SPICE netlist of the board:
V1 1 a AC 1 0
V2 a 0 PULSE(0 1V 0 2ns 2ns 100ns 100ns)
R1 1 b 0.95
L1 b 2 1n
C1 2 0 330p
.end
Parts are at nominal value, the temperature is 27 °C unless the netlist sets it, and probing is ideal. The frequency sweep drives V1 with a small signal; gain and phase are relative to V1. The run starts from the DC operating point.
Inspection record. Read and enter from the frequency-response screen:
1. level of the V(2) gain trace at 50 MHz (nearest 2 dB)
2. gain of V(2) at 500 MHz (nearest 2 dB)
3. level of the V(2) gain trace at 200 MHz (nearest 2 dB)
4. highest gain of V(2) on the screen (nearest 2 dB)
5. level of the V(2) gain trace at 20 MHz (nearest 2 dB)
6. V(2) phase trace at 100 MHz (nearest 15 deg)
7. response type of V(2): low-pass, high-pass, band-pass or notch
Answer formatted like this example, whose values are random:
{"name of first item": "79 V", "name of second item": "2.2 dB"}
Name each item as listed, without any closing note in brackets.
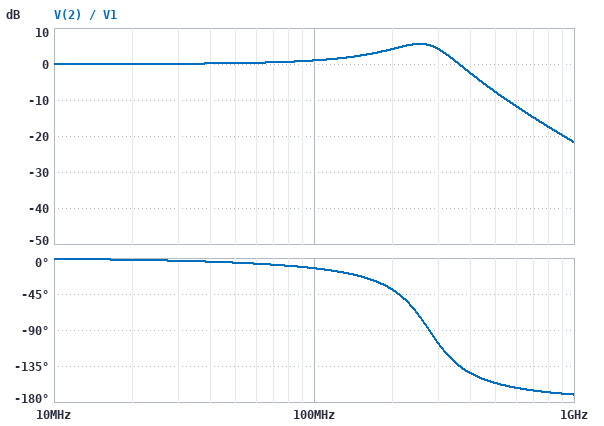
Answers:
{"level of the V(2) gain trace at 50 MHz": "0 dB", "gain of V(2) at 500 MHz": "-8 dB", "level of the V(2) gain trace at 200 MHz": "4 dB", "highest gain of V(2) on the screen": "6 dB", "level of the V(2) gain trace at 20 MHz": "0 dB", "V(2) phase trace at 100 MHz": "-15 deg", "response type of V(2): low-pass, high-pass, band-pass or notch": "low-pass"}
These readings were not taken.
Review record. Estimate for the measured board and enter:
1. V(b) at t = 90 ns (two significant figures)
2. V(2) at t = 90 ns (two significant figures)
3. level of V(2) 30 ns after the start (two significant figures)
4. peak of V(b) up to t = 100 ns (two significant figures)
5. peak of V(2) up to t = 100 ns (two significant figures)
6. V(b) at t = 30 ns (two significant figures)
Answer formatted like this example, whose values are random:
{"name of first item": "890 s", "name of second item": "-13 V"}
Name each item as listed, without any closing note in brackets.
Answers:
{"V(b) at t = 90 ns": "1.0 V", "V(2) at t = 90 ns": "1.0 V", "level of V(2) 30 ns after the start": "1.0 V", "peak of V(b) up to t = 100 ns": "1.1 V", "peak of V(2) up to t = 100 ns": "1.2 V", "V(b) at t = 30 ns": "1.0 V"}
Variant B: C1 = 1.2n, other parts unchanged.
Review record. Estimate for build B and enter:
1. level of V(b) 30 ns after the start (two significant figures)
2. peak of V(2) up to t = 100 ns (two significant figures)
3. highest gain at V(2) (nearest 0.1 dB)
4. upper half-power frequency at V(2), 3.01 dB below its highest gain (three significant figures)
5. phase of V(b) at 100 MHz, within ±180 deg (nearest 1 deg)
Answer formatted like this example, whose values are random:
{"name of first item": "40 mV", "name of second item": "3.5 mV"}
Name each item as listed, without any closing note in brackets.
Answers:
{"level of V(b) 30 ns after the start": "1.0 V", "peak of V(2) up to t = 100 ns": "1.1 V", "highest gain at V(2)": "1.0 dB", "upper half-power frequency at V(2), 3.01 dB below its highest gain": "169 MHz", "phase of V(b) at 100 MHz, within ±180 deg": "-54 deg"}
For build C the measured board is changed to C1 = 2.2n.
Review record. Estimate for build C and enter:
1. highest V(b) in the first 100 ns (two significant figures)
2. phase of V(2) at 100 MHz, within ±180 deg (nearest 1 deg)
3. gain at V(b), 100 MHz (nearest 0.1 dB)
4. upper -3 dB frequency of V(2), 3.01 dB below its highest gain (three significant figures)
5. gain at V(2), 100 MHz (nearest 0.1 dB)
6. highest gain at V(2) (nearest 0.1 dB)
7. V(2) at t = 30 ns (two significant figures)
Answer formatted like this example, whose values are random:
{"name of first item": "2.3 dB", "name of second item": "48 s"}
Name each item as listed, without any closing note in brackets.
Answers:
{"highest V(b) in the first 100 ns": "1.0 V", "phase of V(2) at 100 MHz, within ±180 deg": "-84 deg", "gain at V(b), 100 MHz": "-20.0 dB", "upper -3 dB frequency of V(2), 3.01 dB below its highest gain": "108 MHz", "gain at V(2), 100 MHz": "-2.4 dB", "highest gain at V(2)": "0 dB", "V(2) at t = 30 ns": "1.0 V"}
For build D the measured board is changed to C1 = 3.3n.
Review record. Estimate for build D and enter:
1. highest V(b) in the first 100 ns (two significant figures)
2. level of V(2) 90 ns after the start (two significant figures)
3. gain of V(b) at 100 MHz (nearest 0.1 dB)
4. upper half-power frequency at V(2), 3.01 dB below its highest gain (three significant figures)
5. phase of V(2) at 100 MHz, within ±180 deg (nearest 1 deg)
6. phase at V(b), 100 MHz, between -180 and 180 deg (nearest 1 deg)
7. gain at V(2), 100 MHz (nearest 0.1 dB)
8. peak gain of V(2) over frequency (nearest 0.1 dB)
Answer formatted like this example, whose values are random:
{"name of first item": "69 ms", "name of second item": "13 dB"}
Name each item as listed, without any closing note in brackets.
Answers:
{"highest V(b) in the first 100 ns": "1.0 V", "level of V(2) 90 ns after the start": "1.0 V", "gain of V(b) at 100 MHz": "-16.4 dB", "upper half-power frequency at V(2), 3.01 dB below its highest gain": "69.2 MHz", "phase of V(2) at 100 MHz, within ±180 deg": "-99 deg", "phase at V(b), 100 MHz, between -180 and 180 deg": "81 deg", "gain at V(2), 100 MHz": "-6.0 dB", "peak gain of V(2) over frequency": "0 dB"}
